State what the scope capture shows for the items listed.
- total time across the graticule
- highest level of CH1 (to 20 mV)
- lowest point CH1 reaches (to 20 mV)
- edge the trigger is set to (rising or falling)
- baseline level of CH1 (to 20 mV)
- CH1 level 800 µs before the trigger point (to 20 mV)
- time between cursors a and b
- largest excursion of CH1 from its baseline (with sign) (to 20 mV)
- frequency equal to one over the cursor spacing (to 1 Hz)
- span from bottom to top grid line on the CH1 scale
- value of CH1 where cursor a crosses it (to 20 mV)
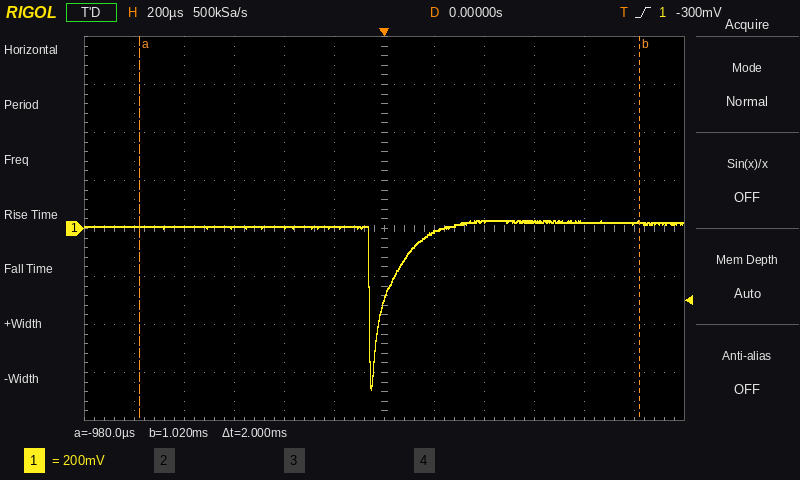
2.4 ms
40 mV
-680 mV
rising
0 mV
0 mV
2 ms
-680 mV
500 Hz
1.6 V
0 mV
